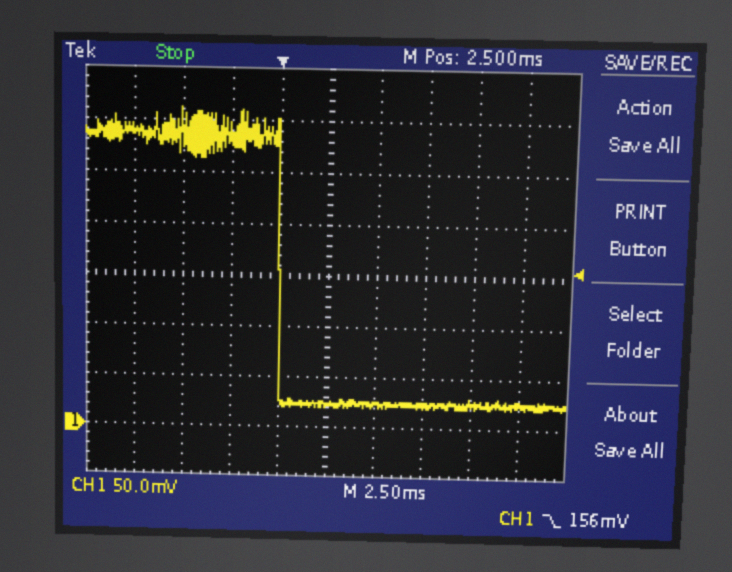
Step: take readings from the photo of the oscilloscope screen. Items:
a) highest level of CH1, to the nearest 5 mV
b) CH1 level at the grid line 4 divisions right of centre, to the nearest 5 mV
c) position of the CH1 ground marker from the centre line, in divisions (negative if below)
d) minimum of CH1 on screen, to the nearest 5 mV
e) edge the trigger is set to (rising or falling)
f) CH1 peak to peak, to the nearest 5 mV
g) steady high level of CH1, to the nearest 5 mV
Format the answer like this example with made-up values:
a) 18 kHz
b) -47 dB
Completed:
a) 310 mV
b) 25 mV
c) -3.0 div
d) 20 mV
e) falling
f) 290 mV
g) 285 mV
